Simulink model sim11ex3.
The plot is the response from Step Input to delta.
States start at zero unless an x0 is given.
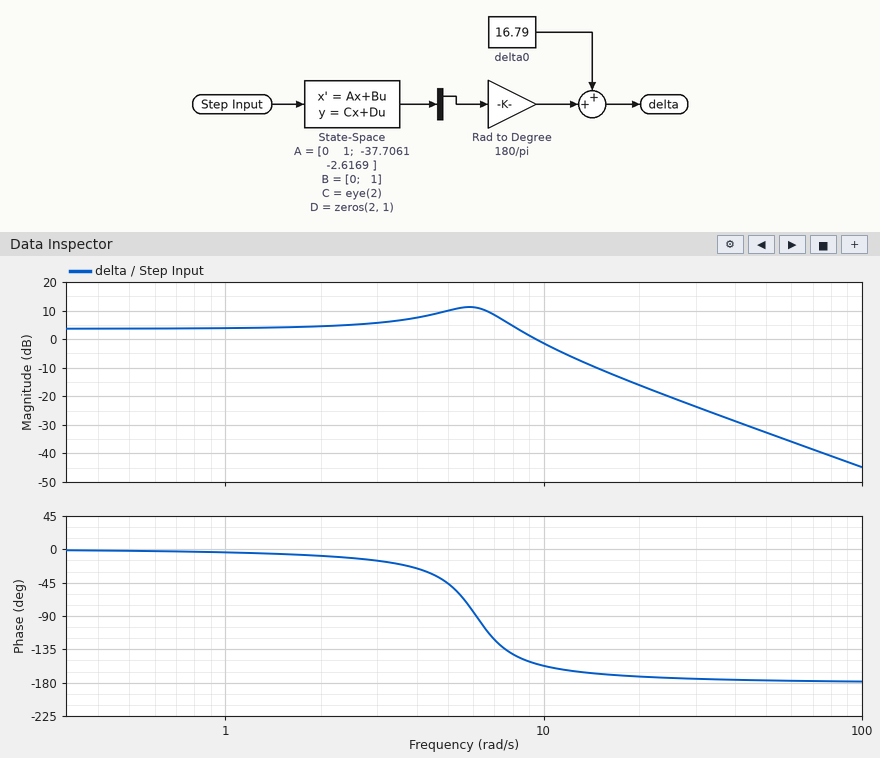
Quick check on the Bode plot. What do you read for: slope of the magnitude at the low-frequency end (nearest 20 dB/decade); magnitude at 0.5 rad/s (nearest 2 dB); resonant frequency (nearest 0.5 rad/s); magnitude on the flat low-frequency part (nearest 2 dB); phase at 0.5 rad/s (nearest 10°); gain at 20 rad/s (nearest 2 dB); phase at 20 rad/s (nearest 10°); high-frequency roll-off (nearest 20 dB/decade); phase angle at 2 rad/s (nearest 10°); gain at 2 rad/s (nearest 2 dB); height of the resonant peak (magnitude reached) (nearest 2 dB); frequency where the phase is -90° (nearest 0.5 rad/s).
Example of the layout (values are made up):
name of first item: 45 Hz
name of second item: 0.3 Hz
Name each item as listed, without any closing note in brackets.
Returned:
slope of the magnitude at the low-frequency end: 0 dB/decade
magnitude at 0.5 rad/s: 4 dB
resonant frequency: 6.0 rad/s
magnitude on the flat low-frequency part: 4 dB
phase at 0.5 rad/s: 0°
gain at 20 rad/s: -16 dB
phase at 20 rad/s: -170°
high-frequency roll-off: -40 dB/decade
phase angle at 2 rad/s: -10°
gain at 2 rad/s: 4 dB
height of the resonant peak (magnitude reached): 12 dB
frequency where the phase is -90°: 6.0 rad/s
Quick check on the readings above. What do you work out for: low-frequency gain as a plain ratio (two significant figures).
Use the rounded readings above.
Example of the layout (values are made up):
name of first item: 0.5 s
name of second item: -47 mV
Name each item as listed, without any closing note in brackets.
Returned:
low-frequency gain as a plain ratio: 1.6
